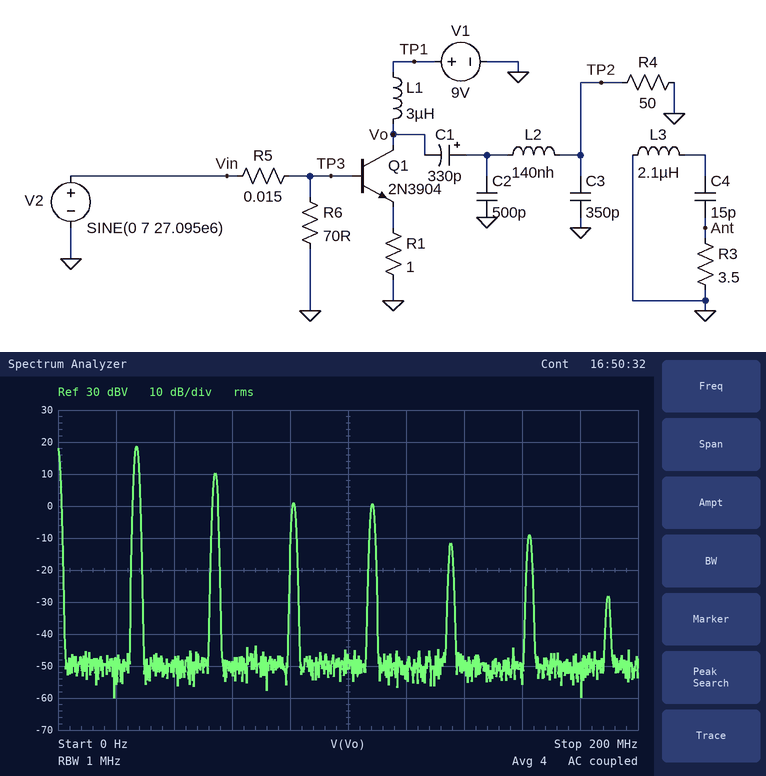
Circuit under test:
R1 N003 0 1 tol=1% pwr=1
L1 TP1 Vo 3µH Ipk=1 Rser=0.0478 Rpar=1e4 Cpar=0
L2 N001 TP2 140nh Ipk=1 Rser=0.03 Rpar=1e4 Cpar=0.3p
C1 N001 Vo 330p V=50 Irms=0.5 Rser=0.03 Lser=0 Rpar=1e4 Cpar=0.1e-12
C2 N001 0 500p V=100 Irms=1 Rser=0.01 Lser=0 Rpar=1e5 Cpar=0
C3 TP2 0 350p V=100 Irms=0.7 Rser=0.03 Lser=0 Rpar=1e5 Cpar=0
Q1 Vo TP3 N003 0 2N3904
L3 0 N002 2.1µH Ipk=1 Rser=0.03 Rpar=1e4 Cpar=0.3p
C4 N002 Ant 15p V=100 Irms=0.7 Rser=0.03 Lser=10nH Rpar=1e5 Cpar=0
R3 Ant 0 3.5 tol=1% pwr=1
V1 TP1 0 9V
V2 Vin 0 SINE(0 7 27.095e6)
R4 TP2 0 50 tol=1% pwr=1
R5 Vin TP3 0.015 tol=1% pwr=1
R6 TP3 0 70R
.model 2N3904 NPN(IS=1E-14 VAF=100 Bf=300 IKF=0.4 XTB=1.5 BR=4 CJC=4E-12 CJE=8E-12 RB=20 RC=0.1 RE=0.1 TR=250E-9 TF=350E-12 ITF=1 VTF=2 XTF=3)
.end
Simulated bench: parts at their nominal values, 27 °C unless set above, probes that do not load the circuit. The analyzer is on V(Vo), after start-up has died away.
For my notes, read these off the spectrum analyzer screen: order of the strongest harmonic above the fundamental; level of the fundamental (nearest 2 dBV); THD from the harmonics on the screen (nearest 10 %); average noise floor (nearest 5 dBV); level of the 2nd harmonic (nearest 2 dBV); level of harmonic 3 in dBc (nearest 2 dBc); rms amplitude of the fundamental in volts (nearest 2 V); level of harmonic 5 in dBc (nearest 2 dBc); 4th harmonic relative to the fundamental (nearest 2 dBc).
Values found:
2
18 dBV
40 %
-50 dBV
10 dBV
-18 dBc
8 V
-30 dBc
-18 dBc
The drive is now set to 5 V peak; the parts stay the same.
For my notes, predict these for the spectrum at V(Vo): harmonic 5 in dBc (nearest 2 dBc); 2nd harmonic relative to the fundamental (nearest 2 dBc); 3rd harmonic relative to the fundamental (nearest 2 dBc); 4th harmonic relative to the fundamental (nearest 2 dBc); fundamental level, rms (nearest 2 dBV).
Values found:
-26 dBc
-12 dBc
-16 dBc
-24 dBc
18 dBV
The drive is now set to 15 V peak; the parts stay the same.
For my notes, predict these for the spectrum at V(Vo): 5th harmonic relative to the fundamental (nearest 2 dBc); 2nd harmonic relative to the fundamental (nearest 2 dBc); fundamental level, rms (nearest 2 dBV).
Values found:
-18 dBc
-4 dBc
20 dBV
